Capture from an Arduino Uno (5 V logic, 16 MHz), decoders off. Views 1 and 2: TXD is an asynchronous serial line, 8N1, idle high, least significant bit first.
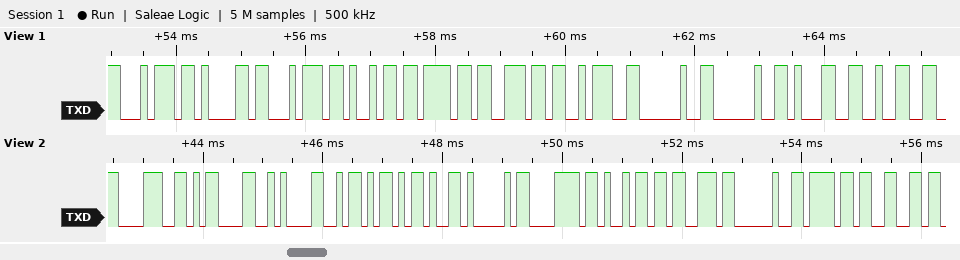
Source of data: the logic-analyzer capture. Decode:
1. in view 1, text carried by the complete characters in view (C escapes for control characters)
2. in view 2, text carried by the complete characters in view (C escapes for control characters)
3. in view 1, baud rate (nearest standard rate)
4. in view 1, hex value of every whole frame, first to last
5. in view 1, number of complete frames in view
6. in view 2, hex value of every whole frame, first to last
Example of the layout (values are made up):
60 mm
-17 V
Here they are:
"tation:  12"
"8\r\nZ-Axis of"
9600 baud
74 61 74 69 6F 6E 3A 20 20 31 32
11
38 0D 0A 5A 2D 41 78 69 73 20 6F 66
